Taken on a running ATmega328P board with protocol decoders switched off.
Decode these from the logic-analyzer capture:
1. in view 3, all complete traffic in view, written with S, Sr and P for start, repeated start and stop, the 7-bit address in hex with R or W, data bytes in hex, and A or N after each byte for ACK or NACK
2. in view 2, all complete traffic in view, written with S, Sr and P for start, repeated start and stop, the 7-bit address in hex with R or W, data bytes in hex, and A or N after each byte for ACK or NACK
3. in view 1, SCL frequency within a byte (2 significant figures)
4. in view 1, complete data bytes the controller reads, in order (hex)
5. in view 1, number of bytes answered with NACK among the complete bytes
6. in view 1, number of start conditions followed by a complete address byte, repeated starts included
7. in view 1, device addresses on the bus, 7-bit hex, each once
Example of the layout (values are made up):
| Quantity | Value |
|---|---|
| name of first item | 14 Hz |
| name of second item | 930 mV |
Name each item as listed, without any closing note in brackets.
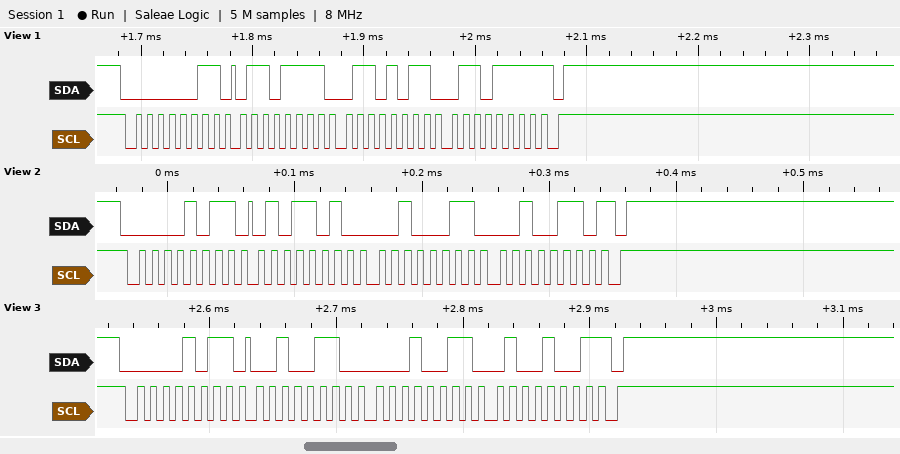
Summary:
| Quantity | Value |
|---|---|
| in view 3, all complete traffic in view, written with S, Sr and P for start, repeated start and stop, the 7-bit address in hex with R or W, data bytes in hex, and A or N after each byte for ACK or NACK | S 05R A 26 A 13 A 49 N P |
| in view 2, all complete traffic in view, written with S, Sr and P for start, repeated start and stop, the 7-bit address in hex with R or W, data bytes in hex, and A or N after each byte for ACK or NACK | S 05R A 5A A 23 A 26 N P |
| in view 1, SCL frequency within a byte | 100 kHz |
| in view 1, complete data bytes the controller reads, in order | 6F 6B 6F |
| in view 1, number of bytes answered with NACK among the complete bytes | 1 |
| in view 1, number of start conditions followed by a complete address byte, repeated starts included | 1 |
| in view 1, device addresses on the bus, 7-bit hex, each once | 0x01 |
